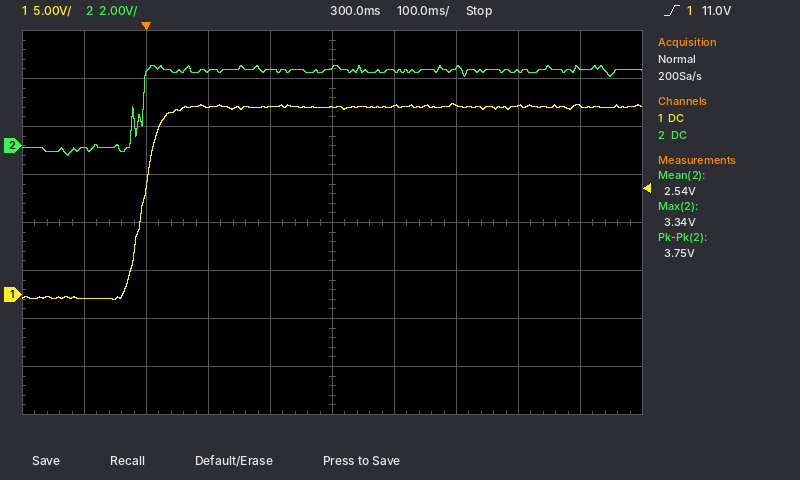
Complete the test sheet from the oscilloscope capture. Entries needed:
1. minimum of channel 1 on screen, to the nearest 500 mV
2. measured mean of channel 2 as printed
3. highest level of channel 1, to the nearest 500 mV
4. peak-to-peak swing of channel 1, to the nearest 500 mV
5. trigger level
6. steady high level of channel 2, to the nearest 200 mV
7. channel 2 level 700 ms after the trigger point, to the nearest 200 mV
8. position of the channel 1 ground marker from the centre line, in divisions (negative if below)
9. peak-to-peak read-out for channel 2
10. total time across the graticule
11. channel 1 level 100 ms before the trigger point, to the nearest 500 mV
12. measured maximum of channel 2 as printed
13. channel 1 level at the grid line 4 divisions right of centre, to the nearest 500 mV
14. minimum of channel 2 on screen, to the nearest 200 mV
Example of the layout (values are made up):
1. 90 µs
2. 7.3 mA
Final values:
1. -500 mV
2. 2.54 V
3. 20.0 V
4. 20.5 V
5. 11.0 V
6. 3.2 V
7. 3.2 V
8. -1.5 div
9. 3.75 V
10. 1 s
11. -500 mV
12. 3.34 V
13. 19.5 V
14. -400 mV
